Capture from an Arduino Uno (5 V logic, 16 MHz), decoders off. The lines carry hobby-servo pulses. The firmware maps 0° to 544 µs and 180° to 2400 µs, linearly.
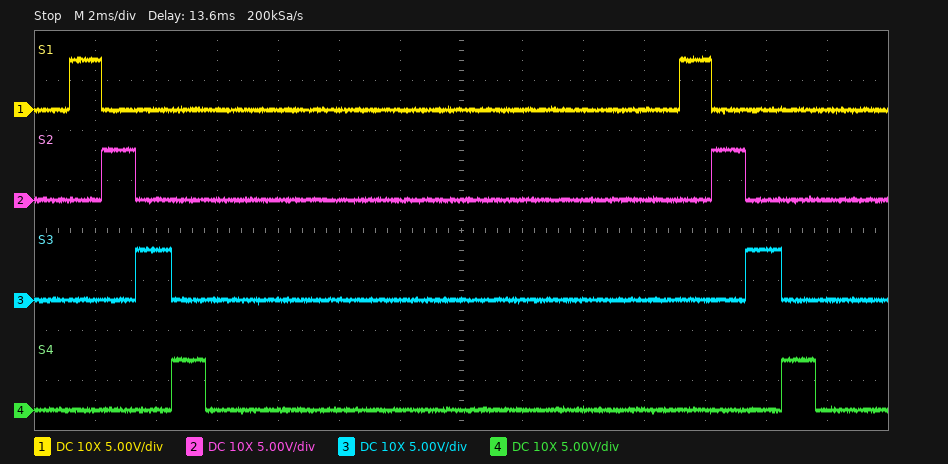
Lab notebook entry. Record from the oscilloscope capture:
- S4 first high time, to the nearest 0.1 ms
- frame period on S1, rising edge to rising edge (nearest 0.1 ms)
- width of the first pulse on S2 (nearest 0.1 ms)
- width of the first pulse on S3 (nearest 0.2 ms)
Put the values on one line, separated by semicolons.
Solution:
1.1 ms; 20.0 ms; 1.1 ms; 1.2 ms
